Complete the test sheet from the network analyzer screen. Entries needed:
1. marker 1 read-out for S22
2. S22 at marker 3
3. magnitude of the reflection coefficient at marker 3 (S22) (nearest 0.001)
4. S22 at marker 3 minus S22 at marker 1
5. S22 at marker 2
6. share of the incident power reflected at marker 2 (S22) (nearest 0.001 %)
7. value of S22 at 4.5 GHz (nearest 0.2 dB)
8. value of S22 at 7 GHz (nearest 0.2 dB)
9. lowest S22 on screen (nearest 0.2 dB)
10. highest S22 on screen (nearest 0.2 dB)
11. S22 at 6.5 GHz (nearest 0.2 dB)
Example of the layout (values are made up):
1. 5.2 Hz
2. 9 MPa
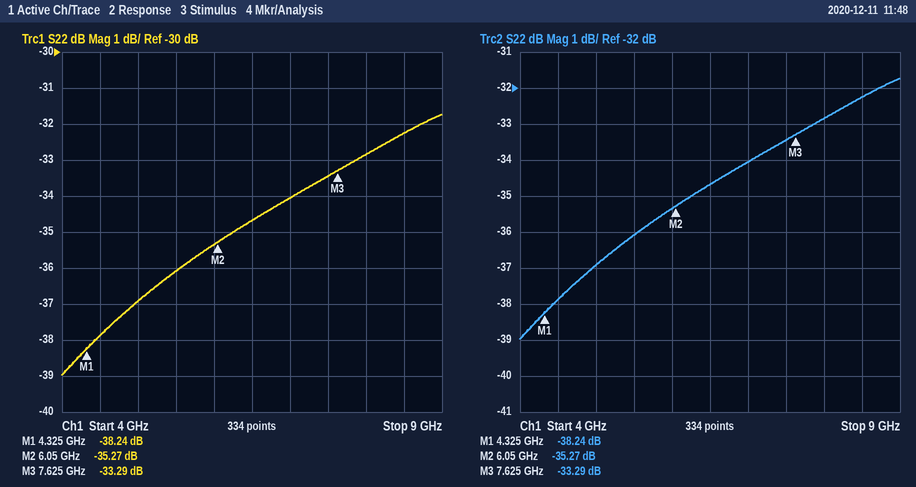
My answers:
1. -38.24 dB
2. -33.29 dB
3. 0.022
4. 4.95 dB
5. -35.27 dB
6. 0.030 %
7. -37.8 dB
8. -34.0 dB
9. -39.0 dB
10. -31.8 dB
11. -34.6 dB
